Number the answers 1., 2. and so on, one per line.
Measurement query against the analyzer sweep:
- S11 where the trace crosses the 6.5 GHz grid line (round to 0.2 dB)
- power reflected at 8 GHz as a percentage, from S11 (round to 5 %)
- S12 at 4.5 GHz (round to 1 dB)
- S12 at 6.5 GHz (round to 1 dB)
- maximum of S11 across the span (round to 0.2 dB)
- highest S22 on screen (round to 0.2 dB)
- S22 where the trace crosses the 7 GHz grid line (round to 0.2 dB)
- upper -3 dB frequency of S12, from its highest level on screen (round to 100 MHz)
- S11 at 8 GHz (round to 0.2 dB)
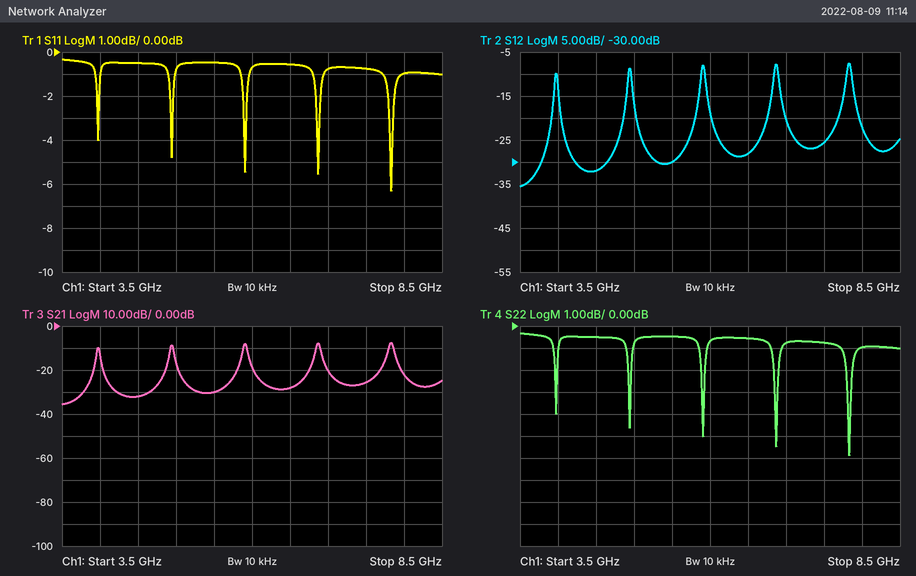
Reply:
1. -0.6 dB
2. 80 %
3. -32 dB
4. -28 dB
5. -0.4 dB
6. -0.4 dB
7. -0.8 dB
8. 7.9 GHz
9. -1.0 dB
